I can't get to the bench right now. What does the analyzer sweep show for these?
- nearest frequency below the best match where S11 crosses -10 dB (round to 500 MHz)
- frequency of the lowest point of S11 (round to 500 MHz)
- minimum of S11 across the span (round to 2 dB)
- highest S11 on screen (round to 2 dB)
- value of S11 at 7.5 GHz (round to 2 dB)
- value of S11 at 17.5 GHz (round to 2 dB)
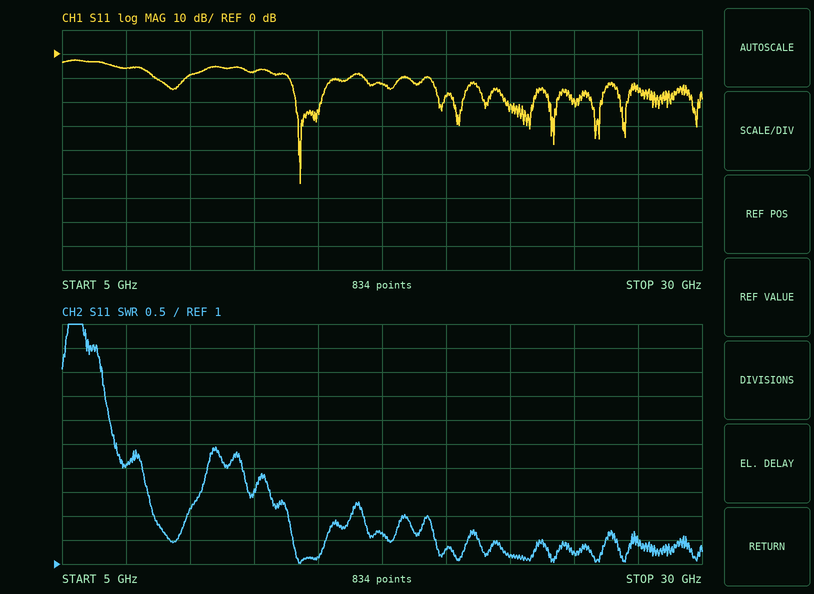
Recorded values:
14.0 GHz
14.5 GHz
-54 dB
-2 dB
-6 dB
-12 dB
